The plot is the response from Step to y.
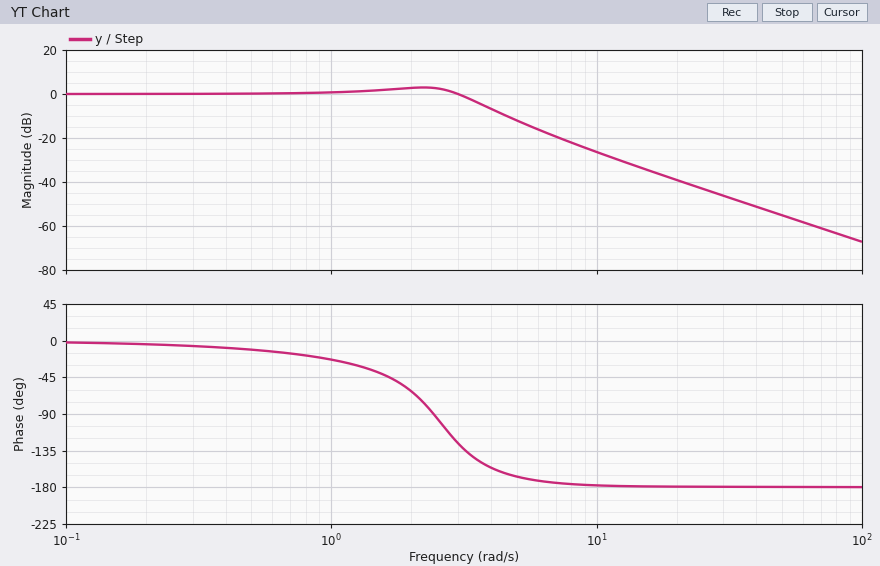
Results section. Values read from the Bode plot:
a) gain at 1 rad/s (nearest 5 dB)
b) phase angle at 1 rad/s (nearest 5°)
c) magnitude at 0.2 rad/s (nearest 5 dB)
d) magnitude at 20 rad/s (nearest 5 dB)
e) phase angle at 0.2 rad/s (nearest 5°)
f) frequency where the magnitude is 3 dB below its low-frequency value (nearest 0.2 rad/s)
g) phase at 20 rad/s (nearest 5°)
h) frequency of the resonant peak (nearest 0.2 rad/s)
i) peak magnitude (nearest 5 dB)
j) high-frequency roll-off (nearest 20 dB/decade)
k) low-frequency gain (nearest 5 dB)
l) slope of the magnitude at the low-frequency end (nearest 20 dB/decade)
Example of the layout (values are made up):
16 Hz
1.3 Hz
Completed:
0 dB
-25°
0 dB
-40 dB
-5°
3.4 rad/s
-180°
2.2 rad/s
5 dB
-40 dB/decade
0 dB
0 dB/decade
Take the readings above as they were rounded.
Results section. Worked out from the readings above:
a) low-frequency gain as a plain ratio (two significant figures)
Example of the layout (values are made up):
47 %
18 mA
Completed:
1.0
